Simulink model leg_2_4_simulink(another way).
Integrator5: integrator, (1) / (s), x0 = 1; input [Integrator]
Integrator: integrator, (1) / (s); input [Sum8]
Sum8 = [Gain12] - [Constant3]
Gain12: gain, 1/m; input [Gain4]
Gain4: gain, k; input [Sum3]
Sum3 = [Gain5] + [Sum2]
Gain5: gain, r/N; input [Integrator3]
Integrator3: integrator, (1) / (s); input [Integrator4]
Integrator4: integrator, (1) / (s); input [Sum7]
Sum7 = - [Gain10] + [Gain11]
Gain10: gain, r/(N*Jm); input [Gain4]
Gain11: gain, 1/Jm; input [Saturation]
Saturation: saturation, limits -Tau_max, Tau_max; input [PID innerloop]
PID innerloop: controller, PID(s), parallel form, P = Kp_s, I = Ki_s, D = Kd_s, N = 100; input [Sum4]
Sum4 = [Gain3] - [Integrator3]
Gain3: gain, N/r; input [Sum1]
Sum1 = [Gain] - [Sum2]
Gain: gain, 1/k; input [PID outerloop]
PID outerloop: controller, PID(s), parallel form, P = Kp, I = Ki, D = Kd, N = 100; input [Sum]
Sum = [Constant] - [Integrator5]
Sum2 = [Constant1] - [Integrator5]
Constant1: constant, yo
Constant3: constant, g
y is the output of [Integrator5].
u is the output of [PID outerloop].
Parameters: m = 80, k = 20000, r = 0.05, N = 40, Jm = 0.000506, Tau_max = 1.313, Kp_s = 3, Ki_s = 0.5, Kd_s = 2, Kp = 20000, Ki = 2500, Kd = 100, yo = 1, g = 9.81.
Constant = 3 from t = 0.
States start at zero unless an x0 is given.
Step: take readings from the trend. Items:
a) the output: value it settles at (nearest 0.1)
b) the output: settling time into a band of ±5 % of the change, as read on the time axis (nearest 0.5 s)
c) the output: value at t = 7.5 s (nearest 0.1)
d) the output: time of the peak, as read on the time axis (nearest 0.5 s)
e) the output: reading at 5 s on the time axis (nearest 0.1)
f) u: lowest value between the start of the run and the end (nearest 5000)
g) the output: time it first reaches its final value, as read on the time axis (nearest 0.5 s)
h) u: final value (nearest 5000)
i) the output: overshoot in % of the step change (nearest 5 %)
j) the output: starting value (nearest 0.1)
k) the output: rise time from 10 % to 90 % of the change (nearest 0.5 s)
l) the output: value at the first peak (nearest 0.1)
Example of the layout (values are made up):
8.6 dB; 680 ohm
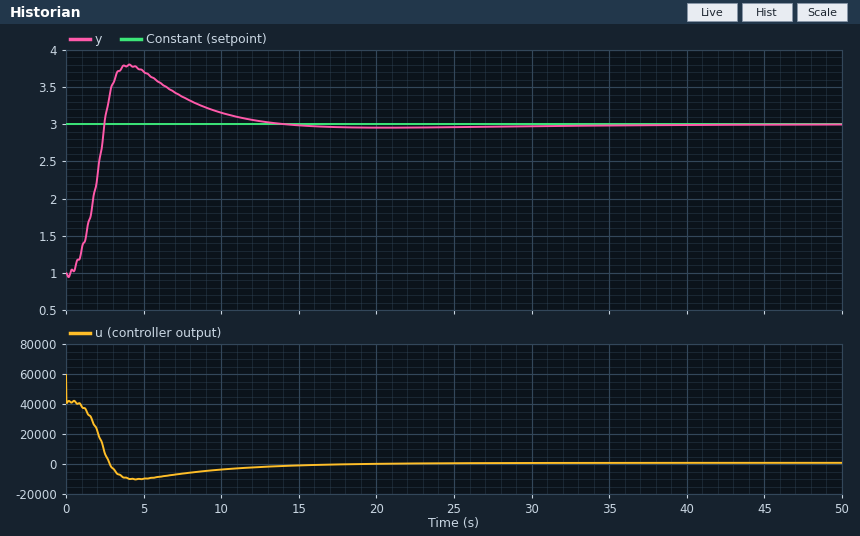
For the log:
3.0; 11.0 s; 3.4; 4.0 s; 3.7; -10000; 2.5 s; 0; 40 %; 1.0; 1.5 s; 3.8
